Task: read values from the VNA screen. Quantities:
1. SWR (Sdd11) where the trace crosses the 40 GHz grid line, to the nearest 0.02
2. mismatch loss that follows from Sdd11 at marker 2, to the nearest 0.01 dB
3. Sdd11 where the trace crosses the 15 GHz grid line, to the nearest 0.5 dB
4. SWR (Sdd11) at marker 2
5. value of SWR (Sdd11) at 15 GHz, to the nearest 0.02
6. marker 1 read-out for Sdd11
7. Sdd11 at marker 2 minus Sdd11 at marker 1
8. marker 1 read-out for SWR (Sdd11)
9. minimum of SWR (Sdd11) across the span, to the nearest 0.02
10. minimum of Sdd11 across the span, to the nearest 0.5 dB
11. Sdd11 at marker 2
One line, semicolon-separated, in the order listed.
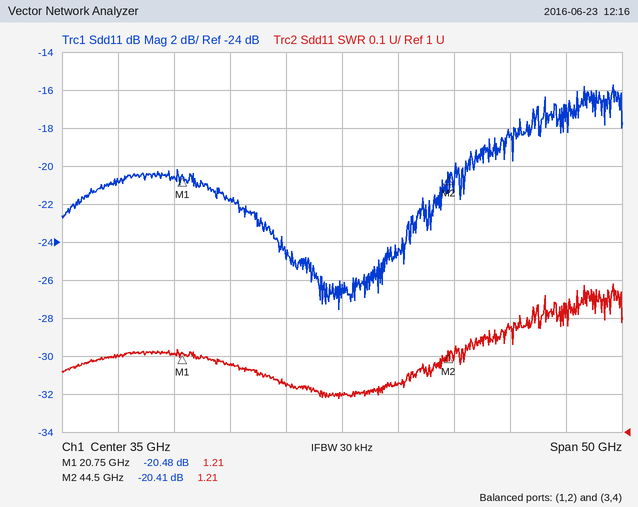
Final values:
1.12; 0.04 dB; -21.0 dB; 1.21; 1.20; -20.48 dB; 0.07 dB; 1.21; 1.08; -27.5 dB; -20.41 dB
